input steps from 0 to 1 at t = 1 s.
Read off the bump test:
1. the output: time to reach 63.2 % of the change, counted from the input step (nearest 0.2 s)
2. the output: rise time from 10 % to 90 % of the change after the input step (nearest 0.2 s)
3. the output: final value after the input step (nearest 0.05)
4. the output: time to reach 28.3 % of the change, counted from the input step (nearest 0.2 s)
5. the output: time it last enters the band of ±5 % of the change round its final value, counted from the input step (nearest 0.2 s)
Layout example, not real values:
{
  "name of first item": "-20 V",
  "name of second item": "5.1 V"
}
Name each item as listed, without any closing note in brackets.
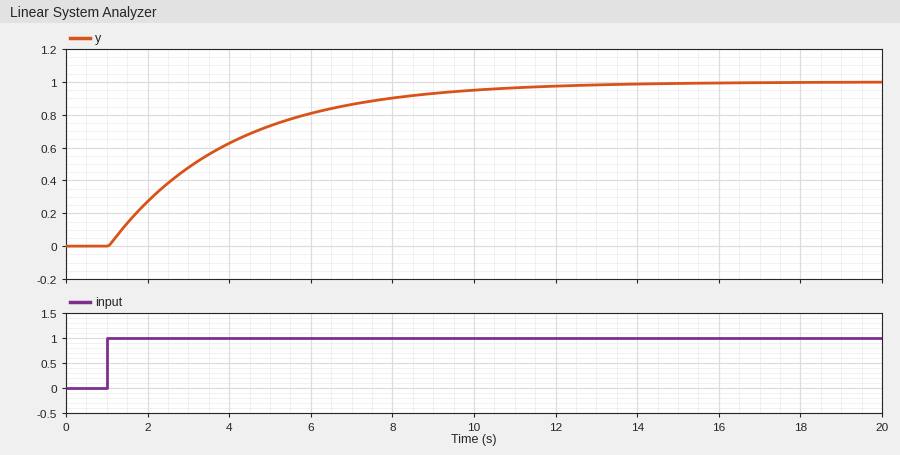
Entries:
{
  "the output: time to reach 63.2 % of the change, counted from the input step": "3.0 s",
  "the output: rise time from 10 % to 90 % of the change after the input step": "6.6 s",
  "the output: final value after the input step": "1.00",
  "the output: time to reach 28.3 % of the change, counted from the input step": "1.0 s",
  "the output: time it last enters the band of ±5 % of the change round its final value, counted from the input step": "9.0 s"
}
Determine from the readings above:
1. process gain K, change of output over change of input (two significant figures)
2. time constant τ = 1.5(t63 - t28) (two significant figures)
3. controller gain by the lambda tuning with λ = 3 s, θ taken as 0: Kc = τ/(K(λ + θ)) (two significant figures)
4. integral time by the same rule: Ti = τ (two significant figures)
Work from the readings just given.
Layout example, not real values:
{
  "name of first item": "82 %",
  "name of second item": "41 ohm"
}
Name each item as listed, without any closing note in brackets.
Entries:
{
  "process gain K, change of output over change of input": "1.0",
  "time constant τ = 1.5(t63 - t28)": "3.0 s",
  "controller gain by the lambda tuning with λ = 3 s, θ taken as 0: Kc = τ/(K(λ + θ))": "1.0",
  "integral time by the same rule: Ti = τ": "3.0 s"
}
